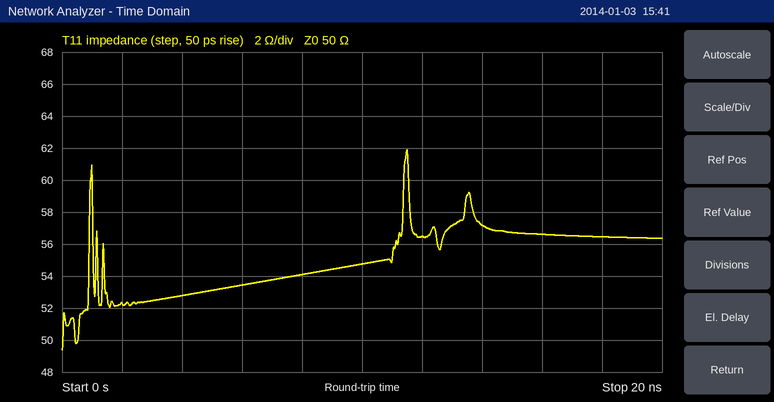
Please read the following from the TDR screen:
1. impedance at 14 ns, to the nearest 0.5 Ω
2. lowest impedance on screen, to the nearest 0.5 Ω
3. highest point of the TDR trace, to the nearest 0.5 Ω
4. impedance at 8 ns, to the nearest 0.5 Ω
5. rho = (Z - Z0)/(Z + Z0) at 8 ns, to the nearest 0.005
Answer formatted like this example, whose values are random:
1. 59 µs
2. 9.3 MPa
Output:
1. 57.0 Ω
2. 49.5 Ω
3. 62.0 Ω
4. 54.0 Ω
5. +0.040
